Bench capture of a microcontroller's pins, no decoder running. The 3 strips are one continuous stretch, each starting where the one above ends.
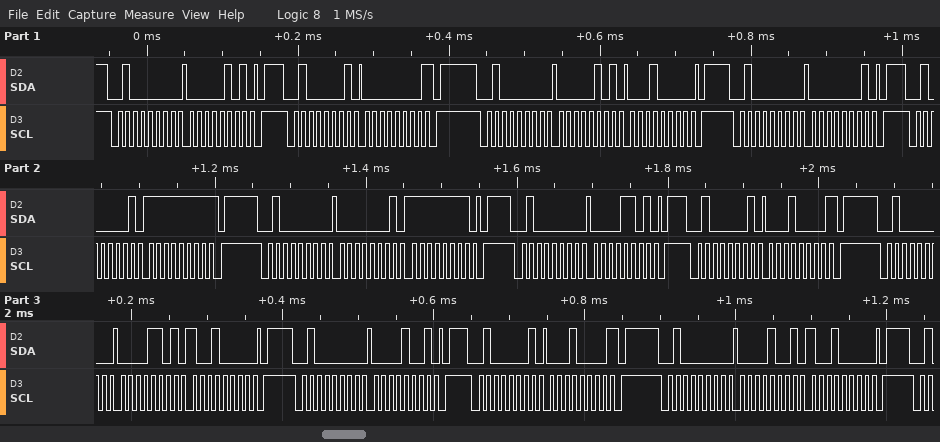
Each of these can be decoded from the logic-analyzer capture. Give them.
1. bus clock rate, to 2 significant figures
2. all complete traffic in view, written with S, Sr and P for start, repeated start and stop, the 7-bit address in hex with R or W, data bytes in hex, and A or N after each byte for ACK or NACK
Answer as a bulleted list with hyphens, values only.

- 100 kHz
- S 20W A 05 A P S 20R A 00 N P S 20W A 05 A 10 A P S 20W A 01 A P S 20R A FF N P S 20W A 01 A FF A P S 20W A 0D A P S 20R A 10 N P S 20W A 0D A 90 A P S 20W A 09 A P S 20R A 10 N P S 20W A 09 A 90 A P
